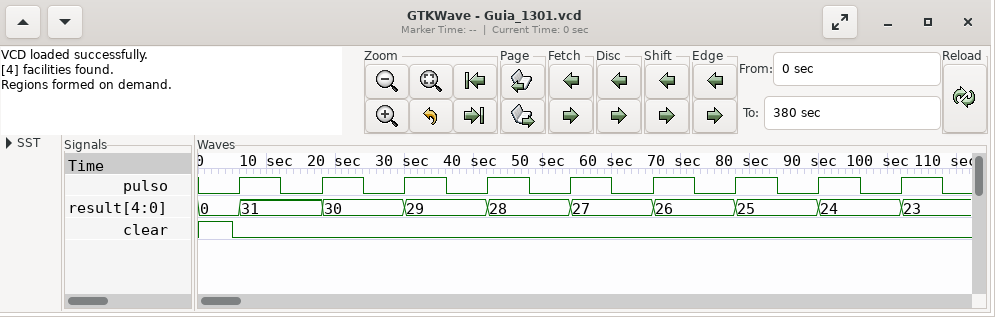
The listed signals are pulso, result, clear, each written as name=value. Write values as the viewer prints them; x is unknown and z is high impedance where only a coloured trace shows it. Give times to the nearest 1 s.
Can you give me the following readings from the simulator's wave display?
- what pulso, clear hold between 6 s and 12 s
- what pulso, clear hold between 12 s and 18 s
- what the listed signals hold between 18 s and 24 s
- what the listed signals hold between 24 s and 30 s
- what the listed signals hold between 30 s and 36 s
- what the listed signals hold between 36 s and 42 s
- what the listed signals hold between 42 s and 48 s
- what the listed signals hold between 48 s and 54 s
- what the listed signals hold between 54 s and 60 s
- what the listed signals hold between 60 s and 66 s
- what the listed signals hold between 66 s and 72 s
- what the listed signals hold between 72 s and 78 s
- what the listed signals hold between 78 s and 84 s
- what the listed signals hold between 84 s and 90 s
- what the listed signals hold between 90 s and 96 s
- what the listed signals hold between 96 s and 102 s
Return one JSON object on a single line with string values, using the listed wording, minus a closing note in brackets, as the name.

{"what pulso, clear hold between 6 s and 12 s": "pulso=1, clear=0", "what pulso, clear hold between 12 s and 18 s": "pulso=0, clear=0", "what the listed signals hold between 18 s and 24 s": "pulso=1, result=30, clear=0", "what the listed signals hold between 24 s and 30 s": "pulso=0, result=30, clear=0", "what the listed signals hold between 30 s and 36 s": "pulso=1, result=29, clear=0", "what the listed signals hold between 36 s and 42 s": "pulso=0, result=29, clear=0", "what the listed signals hold between 42 s and 48 s": "pulso=1, result=28, clear=0", "what the listed signals hold between 48 s and 54 s": "pulso=0, result=28, clear=0", "what the listed signals hold between 54 s and 60 s": "pulso=1, result=27, clear=0", "what the listed signals hold between 60 s and 66 s": "pulso=0, result=27, clear=0", "what the listed signals hold between 66 s and 72 s": "pulso=1, result=26, clear=0", "what the listed signals hold between 72 s and 78 s": "pulso=0, result=26, clear=0", "what the listed signals hold between 78 s and 84 s": "pulso=1, result=25, clear=0", "what the listed signals hold between 84 s and 90 s": "pulso=0, result=25, clear=0", "what the listed signals hold between 90 s and 96 s": "pulso=1, result=24, clear=0", "what the listed signals hold between 96 s and 102 s": "pulso=0, result=24, clear=0"}
